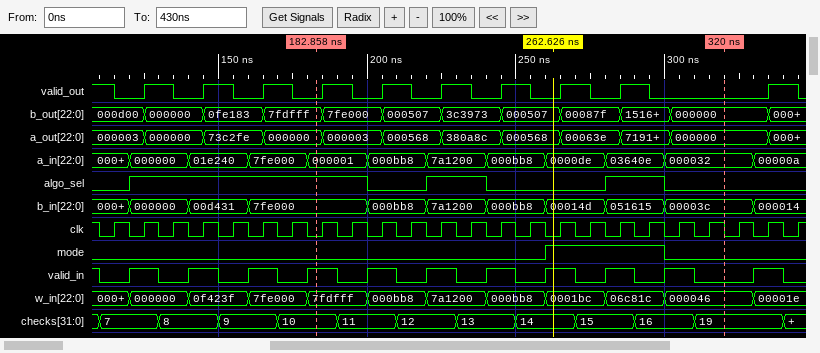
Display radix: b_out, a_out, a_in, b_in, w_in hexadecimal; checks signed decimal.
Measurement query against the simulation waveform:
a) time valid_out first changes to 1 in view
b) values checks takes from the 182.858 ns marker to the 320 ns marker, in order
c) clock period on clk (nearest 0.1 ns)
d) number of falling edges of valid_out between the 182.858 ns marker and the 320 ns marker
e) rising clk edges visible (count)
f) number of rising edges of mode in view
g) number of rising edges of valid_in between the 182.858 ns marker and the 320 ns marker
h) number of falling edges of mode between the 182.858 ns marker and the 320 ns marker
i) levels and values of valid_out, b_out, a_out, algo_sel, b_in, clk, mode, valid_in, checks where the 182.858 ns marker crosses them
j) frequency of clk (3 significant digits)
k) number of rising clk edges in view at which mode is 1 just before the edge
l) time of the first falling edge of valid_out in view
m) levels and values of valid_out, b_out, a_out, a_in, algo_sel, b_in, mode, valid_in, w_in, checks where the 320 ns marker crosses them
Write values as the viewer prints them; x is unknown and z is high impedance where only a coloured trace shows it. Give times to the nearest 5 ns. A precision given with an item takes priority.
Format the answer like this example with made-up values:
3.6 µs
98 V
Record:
125 ns
10, 11, 12, 13, 14, 15, 16, 19
10 ns
6
24
1
6
1
valid_out=0, b_out=7fdfff, a_out=000000, algo_sel=1, b_in=7fe000, clk=0, mode=0, valid_in=1, checks=10
100 MHz
4
115 ns
valid_out=0, b_out=000000, a_out=000000, a_in=000032, algo_sel=0, b_in=00003c, mode=0, valid_in=0, w_in=000046, checks=19
